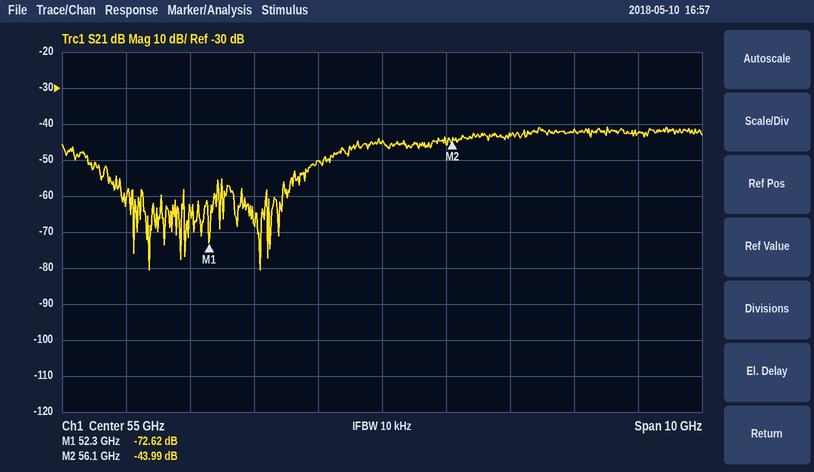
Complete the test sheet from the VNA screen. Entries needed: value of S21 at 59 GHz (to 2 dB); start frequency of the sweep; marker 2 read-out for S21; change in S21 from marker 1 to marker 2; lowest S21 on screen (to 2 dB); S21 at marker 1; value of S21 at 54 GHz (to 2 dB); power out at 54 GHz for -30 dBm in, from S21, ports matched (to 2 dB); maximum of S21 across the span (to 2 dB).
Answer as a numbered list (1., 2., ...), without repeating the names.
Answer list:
1. -42 dB
2. 50 GHz
3. -43.99 dB
4. 28.63 dB
5. -80 dB
6. -72.62 dB
7. -50 dB
8. -80 dBm
9. -40 dB
